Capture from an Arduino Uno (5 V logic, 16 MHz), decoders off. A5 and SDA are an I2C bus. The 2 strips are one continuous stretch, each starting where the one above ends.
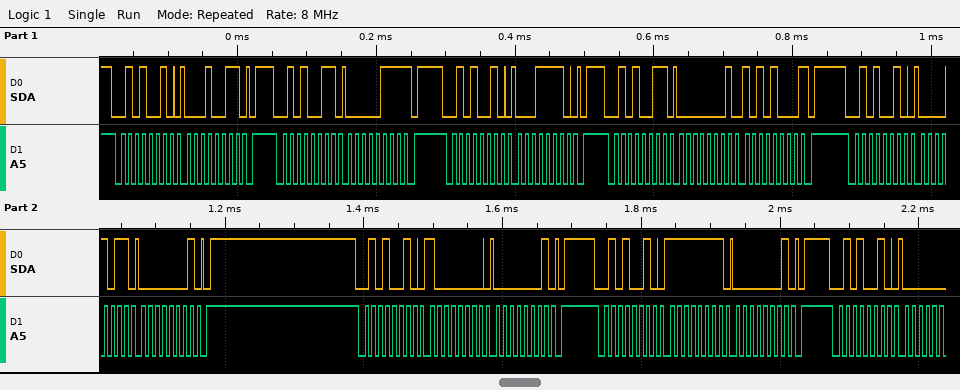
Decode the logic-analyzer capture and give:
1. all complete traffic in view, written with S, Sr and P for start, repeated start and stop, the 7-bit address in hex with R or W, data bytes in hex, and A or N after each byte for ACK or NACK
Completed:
S 29W A 13 A P S 29R A 07 N P S 29W A 1E A P S 29R A 01 A A8 N P S 29W A 0B A 01 A P S 29W A 80 A 01 A P S 29W A FF A 01 A P S 29W A
